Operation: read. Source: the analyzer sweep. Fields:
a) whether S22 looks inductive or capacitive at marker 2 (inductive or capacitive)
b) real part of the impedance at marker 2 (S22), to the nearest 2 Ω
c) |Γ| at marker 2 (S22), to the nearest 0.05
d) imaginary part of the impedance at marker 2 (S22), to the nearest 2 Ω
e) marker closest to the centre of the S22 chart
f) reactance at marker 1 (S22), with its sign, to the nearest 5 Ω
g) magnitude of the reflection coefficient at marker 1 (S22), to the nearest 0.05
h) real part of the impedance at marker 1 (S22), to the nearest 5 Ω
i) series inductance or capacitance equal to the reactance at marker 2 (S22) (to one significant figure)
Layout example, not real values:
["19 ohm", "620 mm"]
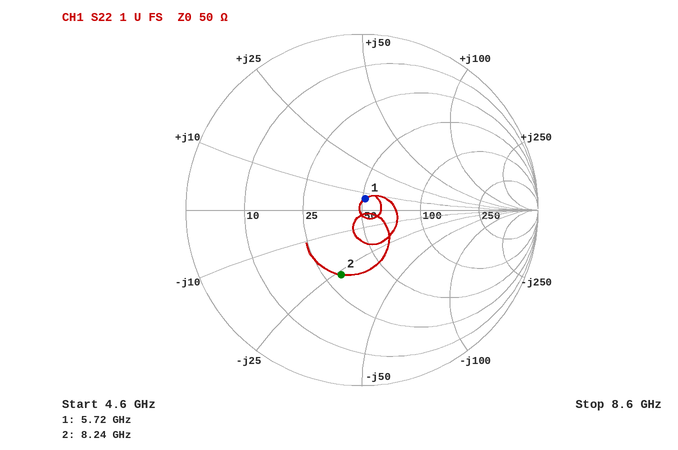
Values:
["capacitive", "30 Ω", "0.40", "-26 Ω", "marker 1", "+5 Ω", "0.05", "50 Ω", "700 fF"]
